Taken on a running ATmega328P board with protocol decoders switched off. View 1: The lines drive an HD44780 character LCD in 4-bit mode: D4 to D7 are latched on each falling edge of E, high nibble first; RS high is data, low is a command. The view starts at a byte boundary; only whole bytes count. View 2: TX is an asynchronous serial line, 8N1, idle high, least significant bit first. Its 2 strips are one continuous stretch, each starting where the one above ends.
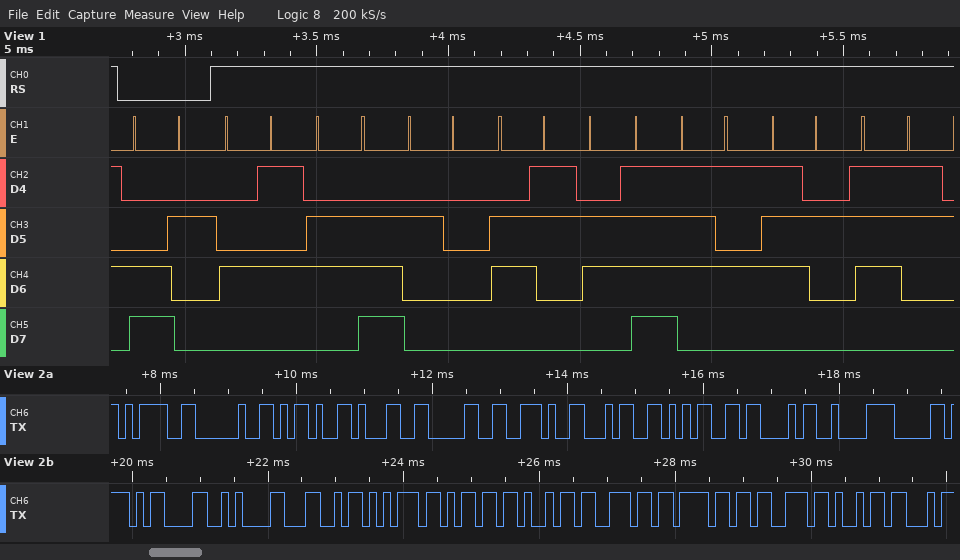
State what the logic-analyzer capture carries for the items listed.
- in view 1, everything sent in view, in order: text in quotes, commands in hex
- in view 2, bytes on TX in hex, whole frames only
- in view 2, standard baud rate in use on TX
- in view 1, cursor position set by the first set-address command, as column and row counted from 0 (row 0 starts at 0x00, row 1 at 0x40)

0xC2 "En cours"
3D 20 2D 31 30 2E 34 35 43 C2 B0 0D 0A 4C 75 6D 69 6E 6F 73 69
9600 baud
column 2, row 1
